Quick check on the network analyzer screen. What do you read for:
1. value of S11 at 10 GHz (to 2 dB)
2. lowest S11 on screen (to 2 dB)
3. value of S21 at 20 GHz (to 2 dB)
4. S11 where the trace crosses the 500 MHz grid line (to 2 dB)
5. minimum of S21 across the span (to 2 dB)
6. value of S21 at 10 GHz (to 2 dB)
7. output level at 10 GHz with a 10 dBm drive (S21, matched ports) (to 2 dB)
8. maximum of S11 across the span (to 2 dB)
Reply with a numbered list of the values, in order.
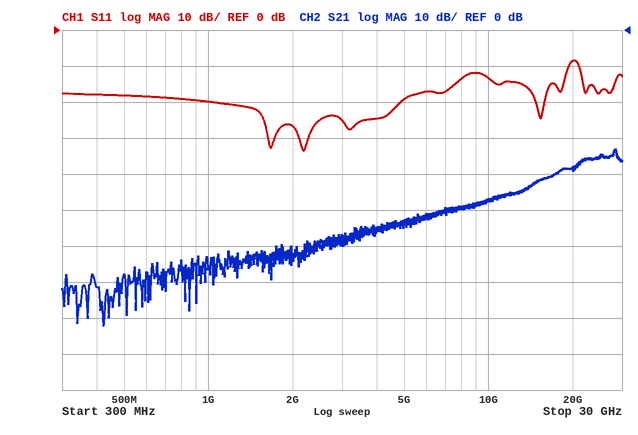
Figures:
1. -14 dB
2. -34 dB
3. -38 dB
4. -18 dB
5. -82 dB
6. -48 dB
7. -38 dBm
8. -8 dB
